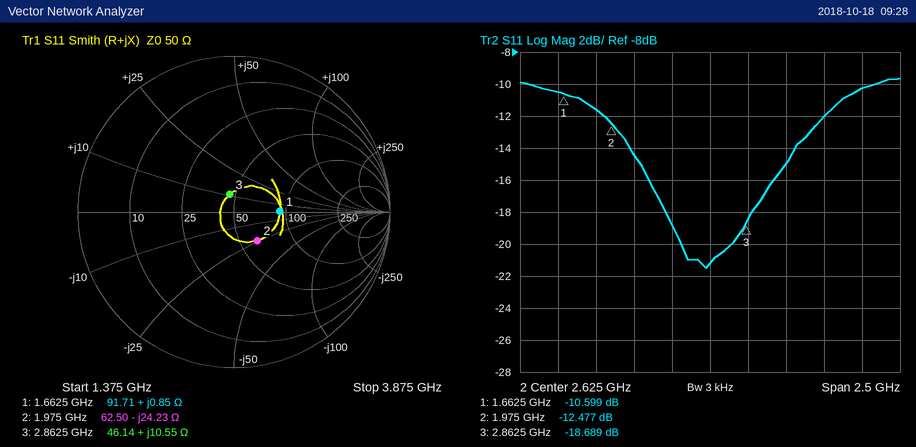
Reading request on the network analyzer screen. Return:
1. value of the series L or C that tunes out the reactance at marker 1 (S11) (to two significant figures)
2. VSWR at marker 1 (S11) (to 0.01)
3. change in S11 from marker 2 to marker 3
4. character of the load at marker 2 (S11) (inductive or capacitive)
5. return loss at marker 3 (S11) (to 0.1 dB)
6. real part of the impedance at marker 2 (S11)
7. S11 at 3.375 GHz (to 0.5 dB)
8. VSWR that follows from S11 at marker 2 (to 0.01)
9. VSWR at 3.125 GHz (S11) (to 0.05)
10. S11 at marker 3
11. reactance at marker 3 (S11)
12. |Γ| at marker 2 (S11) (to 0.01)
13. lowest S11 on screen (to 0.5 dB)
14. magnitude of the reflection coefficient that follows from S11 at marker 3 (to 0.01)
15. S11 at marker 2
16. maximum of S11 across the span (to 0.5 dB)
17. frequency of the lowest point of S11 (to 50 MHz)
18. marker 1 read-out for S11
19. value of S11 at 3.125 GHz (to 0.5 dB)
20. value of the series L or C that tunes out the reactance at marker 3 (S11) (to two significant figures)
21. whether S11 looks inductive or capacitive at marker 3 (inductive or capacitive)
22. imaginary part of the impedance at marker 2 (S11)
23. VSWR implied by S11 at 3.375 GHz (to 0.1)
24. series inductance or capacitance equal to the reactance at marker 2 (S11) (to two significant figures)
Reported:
110 pF
1.84
-6.212 dB
capacitive
18.7 dB
62.50 Ω
-12.0 dB
1.62
1.45
-18.689 dB
+10.55 Ω
0.24
-21.5 dB
0.12
-12.477 dB
-9.5 dB
2.60 GHz
-10.599 dB
-15.0 dB
5.3 pF
inductive
-24.23 Ω
1.7
3.3 pF
